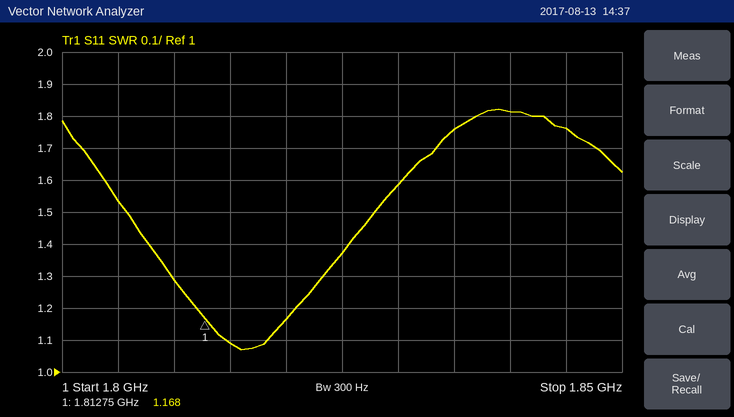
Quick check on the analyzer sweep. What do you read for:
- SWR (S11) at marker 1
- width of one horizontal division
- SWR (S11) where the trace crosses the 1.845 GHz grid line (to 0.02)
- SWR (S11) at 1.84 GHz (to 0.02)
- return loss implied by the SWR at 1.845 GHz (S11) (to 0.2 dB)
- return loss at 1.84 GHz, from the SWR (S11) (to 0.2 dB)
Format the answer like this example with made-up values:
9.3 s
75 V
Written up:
1.168
5 MHz
1.76
1.82
11.2 dB
10.8 dB
